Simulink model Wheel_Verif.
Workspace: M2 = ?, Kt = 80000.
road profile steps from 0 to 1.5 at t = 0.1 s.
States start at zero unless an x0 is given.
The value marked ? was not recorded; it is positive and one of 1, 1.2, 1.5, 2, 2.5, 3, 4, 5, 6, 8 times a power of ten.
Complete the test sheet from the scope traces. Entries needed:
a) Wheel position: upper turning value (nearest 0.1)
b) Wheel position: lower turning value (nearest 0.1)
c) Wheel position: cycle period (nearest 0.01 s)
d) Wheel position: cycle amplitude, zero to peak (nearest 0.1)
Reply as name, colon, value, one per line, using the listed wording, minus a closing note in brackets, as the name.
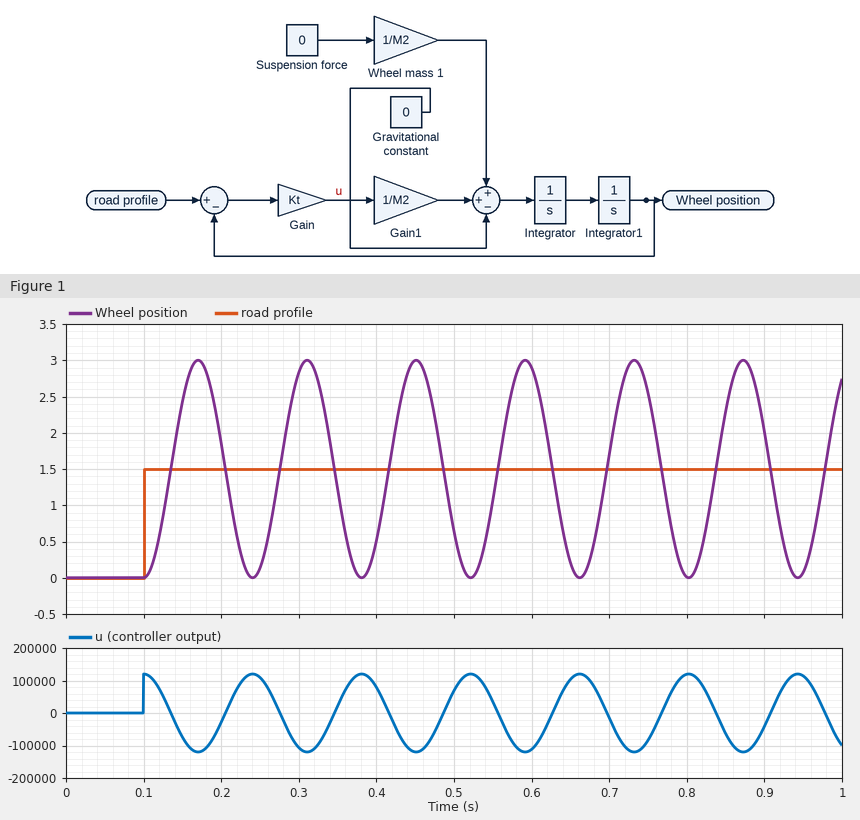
Wheel position: upper turning value: 3.0
Wheel position: lower turning value: 0.0
Wheel position: cycle period: 0.14 s
Wheel position: cycle amplitude, zero to peak: 1.5
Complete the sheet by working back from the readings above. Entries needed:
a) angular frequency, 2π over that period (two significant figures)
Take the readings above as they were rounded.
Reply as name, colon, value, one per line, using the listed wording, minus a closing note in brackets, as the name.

angular frequency, 2π over that period: 45 rad/s
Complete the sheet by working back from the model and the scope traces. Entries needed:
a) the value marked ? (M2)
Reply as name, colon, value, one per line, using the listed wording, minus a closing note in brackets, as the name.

the value marked ?: 40
